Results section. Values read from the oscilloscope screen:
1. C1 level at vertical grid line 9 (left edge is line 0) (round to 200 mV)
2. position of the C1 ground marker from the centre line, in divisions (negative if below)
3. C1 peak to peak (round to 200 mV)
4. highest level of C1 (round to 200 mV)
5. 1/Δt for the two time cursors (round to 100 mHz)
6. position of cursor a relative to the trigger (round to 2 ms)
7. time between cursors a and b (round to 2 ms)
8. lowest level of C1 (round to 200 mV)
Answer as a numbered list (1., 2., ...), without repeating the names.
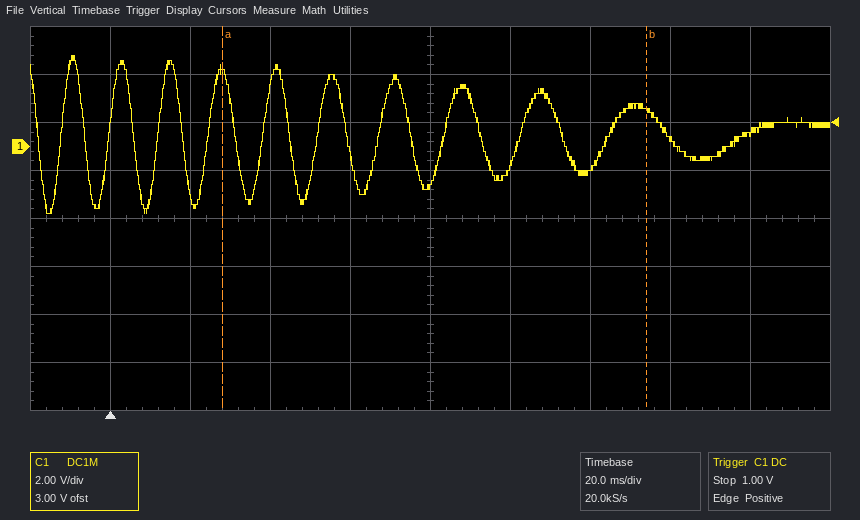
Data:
1. 600 mV
2. +1.5 div
3. 6.6 V
4. 3.8 V
5. 9.4 Hz
6. +28 ms
7. 106 ms
8. -2.8 V
